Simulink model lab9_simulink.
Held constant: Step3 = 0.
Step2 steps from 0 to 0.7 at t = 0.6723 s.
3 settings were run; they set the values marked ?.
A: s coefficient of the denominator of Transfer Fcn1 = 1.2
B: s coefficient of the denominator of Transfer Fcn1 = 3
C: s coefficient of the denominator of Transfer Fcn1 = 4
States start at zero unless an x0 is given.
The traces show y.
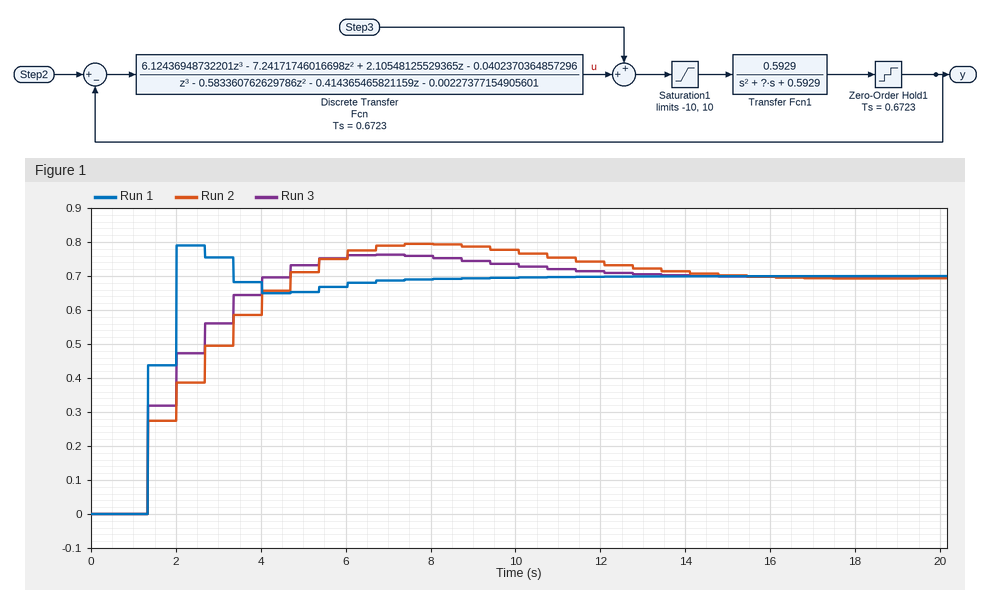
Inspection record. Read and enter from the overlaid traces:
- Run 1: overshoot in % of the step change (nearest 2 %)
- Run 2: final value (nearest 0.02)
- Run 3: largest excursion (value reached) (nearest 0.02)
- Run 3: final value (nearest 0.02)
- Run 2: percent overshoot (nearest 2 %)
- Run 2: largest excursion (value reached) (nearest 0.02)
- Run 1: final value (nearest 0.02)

12 %
0.70
0.76
0.70
14 %
0.80
0.70
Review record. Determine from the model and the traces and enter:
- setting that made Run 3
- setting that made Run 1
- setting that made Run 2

B
A
C
